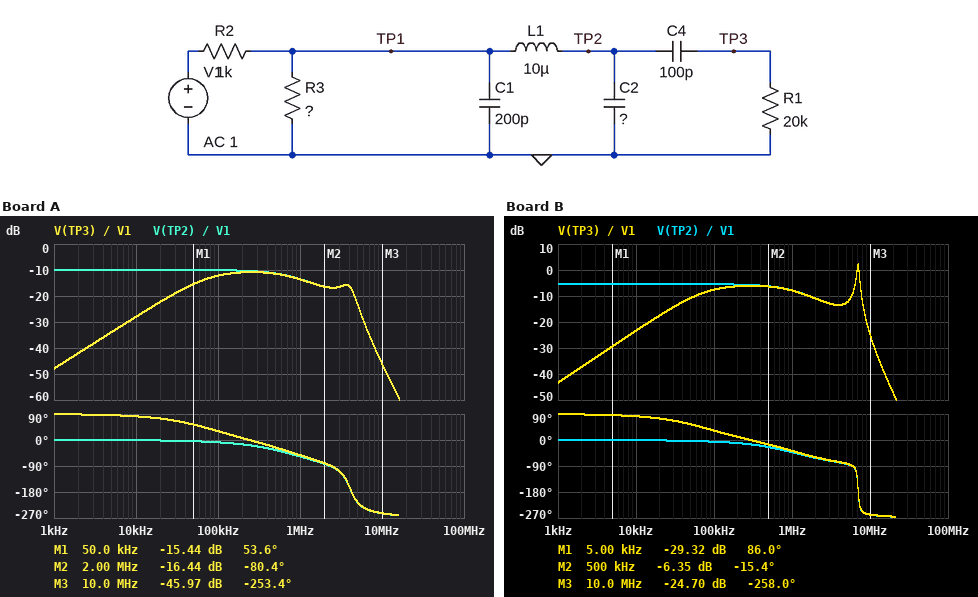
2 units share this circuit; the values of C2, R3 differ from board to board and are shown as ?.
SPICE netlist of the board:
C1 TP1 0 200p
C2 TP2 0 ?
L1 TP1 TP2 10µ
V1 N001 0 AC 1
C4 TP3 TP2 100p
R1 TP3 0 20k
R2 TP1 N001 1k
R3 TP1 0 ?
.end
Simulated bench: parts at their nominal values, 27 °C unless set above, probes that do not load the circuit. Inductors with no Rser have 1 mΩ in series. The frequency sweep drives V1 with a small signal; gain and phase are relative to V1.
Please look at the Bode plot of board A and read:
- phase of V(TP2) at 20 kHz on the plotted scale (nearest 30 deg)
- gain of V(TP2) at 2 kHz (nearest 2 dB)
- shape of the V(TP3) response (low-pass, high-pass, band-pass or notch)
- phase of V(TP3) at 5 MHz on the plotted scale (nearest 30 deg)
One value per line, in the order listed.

0 deg
-10 dB
band-pass
-210 deg
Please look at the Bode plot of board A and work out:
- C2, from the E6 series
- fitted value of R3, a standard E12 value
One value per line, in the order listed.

470 pF
470 Ω
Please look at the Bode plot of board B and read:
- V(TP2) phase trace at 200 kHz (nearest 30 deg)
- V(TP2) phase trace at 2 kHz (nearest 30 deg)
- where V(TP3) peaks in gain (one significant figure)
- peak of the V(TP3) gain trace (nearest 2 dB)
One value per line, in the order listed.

0 deg
0 deg
7 MHz
2 dB
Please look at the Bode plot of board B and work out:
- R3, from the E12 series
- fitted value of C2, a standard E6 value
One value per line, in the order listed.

1.2 kΩ
68 pF
